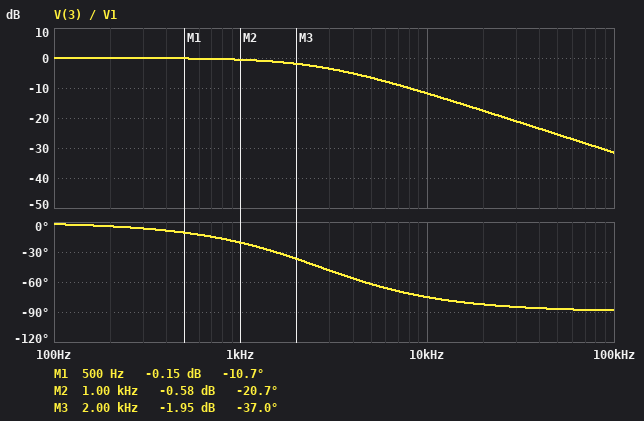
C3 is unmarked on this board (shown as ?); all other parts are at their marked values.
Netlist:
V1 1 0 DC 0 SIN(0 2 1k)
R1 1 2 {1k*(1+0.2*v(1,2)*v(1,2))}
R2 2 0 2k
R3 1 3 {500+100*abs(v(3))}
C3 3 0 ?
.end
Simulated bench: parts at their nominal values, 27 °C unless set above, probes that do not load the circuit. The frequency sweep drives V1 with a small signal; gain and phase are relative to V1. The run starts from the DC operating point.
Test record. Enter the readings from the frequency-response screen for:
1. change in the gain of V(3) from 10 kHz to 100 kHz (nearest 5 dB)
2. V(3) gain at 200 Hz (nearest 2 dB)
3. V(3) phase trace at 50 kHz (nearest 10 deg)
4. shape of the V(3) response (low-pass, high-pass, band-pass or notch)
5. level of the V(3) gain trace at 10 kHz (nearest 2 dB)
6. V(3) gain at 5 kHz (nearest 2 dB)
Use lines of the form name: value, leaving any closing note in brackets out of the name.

change in the gain of V(3) from 10 kHz to 100 kHz: -20 dB
V(3) gain at 200 Hz: 0 dB
V(3) phase trace at 50 kHz: -90 deg
shape of the V(3) response: low-pass
level of the V(3) gain trace at 10 kHz: -12 dB
V(3) gain at 5 kHz: -6 dB
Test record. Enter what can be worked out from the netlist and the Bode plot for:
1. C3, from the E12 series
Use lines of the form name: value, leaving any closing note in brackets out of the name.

C3, from the E12 series: 120 nF
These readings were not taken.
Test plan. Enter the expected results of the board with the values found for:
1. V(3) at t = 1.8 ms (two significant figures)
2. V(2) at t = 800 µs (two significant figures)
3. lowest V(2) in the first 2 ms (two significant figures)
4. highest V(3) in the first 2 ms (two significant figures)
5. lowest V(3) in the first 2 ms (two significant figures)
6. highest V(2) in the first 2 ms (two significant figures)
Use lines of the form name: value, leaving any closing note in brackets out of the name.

V(3) at t = 1.8 ms: -1.8 V
V(2) at t = 800 µs: -1.2 V
lowest V(2) in the first 2 ms: -1.3 V
highest V(3) in the first 2 ms: 1.8 V
lowest V(3) in the first 2 ms: -1.8 V
highest V(2) in the first 2 ms: 1.3 V
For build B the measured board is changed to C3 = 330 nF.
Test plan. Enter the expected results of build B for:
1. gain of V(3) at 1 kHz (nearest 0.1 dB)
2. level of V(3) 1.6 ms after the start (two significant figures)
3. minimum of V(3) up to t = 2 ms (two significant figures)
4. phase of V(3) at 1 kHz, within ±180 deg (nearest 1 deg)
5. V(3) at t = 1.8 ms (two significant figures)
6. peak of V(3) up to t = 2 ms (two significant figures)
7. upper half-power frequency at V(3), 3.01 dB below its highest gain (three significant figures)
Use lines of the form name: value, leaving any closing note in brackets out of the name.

gain of V(3) at 1 kHz: -3.2 dB
level of V(3) 1.6 ms after the start: 310 mV
minimum of V(3) up to t = 2 ms: -1.3 V
phase of V(3) at 1 kHz, within ±180 deg: -46 deg
V(3) at t = 1.8 ms: -1.1 V
peak of V(3) up to t = 2 ms: 1.4 V
upper half-power frequency at V(3), 3.01 dB below its highest gain: 965 Hz
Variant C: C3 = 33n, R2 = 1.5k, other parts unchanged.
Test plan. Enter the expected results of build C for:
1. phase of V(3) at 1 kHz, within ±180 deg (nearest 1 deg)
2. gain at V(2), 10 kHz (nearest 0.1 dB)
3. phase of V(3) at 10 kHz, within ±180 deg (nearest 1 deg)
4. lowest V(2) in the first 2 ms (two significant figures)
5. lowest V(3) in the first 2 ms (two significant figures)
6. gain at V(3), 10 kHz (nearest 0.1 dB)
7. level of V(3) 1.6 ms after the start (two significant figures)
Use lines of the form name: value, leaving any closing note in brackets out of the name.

phase of V(3) at 1 kHz, within ±180 deg: -6 deg
gain at V(2), 10 kHz: -4.4 dB
phase of V(3) at 10 kHz, within ±180 deg: -46 deg
lowest V(2) in the first 2 ms: -1.1 V
lowest V(3) in the first 2 ms: -2.0 V
gain at V(3), 10 kHz: -3.2 dB
level of V(3) 1.6 ms after the start: -970 mV
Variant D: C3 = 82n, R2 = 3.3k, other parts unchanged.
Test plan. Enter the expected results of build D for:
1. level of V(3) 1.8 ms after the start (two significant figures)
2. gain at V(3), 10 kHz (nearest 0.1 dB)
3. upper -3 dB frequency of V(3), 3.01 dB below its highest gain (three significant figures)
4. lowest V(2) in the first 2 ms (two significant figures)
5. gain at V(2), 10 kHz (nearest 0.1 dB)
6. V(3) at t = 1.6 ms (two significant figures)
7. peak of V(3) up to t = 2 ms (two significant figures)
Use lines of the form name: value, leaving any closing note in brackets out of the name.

level of V(3) 1.8 ms after the start: -1.9 V
gain at V(3), 10 kHz: -8.8 dB
upper -3 dB frequency of V(3), 3.01 dB below its highest gain: 3.88 kHz
lowest V(2) in the first 2 ms: -1.5 V
gain at V(2), 10 kHz: -2.3 dB
V(3) at t = 1.6 ms: -670 mV
peak of V(3) up to t = 2 ms: 1.9 V
